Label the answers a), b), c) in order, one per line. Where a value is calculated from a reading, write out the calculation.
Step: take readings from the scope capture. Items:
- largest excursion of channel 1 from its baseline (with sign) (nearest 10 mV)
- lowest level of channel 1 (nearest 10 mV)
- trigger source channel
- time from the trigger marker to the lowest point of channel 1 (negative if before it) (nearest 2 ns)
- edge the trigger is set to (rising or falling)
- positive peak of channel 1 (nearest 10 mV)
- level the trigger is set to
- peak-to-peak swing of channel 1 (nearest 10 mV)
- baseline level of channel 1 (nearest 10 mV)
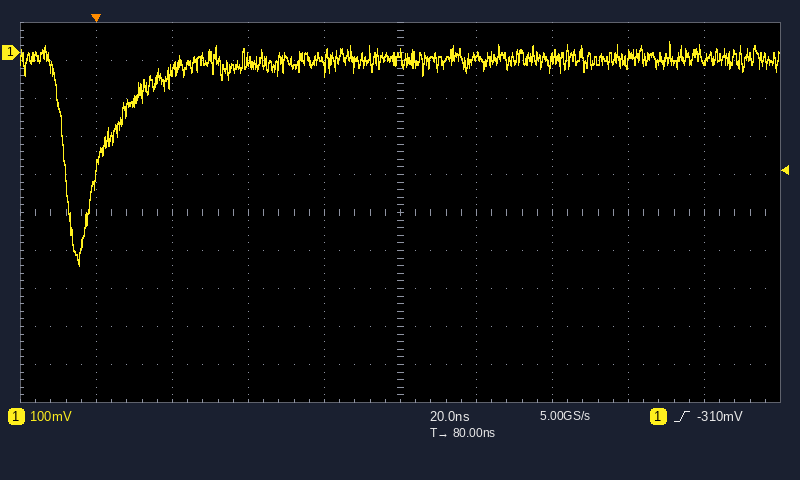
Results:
a) -560 mV − (-20 mV) = -540 mV
b) -560 mV
c) channel 1
d) -4 ns
e) rising
f) 30 mV
g) -310 mV
h) 30 mV − (-560 mV) = 590 mV
i) -20 mV
